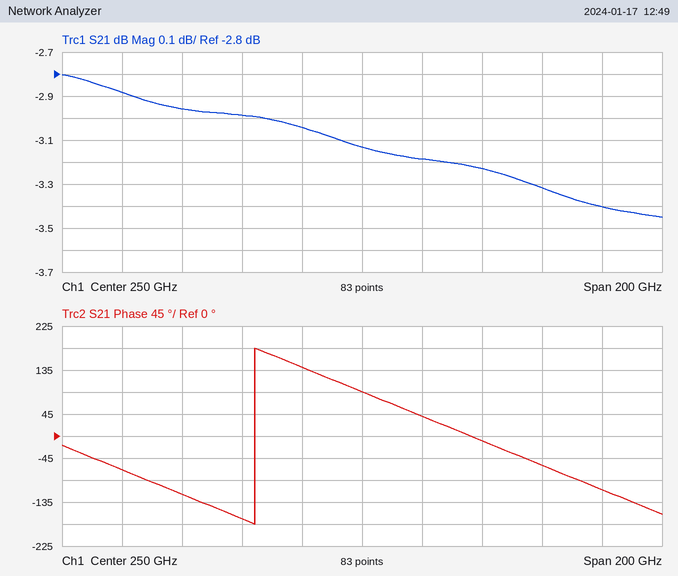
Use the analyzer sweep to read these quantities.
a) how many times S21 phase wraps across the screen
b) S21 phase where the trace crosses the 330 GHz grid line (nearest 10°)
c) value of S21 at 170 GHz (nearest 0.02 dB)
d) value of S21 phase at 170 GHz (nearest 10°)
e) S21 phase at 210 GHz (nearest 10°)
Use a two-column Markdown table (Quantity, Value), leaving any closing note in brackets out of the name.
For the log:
| Quantity | Value |
|---|---|
| how many times S21 phase wraps across the screen | 1 |
| S21 phase where the trace crosses the 330 GHz grid line | -110° |
| value of S21 at 170 GHz | -2.88 dB |
| value of S21 phase at 170 GHz | -70° |
| S21 phase at 210 GHz | -170° |
